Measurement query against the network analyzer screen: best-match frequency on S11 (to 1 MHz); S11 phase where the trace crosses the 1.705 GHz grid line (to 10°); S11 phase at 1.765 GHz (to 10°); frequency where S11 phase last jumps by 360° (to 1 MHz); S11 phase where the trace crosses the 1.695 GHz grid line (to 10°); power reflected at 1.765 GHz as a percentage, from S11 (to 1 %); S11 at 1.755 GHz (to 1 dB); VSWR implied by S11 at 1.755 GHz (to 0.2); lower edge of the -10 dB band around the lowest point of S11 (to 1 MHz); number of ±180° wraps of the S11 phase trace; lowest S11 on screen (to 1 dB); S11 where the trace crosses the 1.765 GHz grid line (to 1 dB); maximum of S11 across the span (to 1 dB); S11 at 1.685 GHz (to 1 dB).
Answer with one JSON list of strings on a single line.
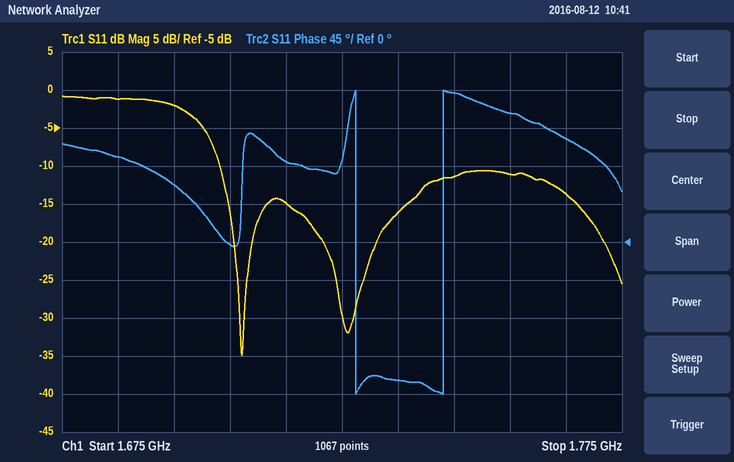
["1.707 GHz", "0°", "120°", "1.743 GHz", "70°", "4 %", "-11 dB", "1.8", "1.703 GHz", "2", "-35 dB", "-14 dB", "-1 dB", "-1 dB"]
